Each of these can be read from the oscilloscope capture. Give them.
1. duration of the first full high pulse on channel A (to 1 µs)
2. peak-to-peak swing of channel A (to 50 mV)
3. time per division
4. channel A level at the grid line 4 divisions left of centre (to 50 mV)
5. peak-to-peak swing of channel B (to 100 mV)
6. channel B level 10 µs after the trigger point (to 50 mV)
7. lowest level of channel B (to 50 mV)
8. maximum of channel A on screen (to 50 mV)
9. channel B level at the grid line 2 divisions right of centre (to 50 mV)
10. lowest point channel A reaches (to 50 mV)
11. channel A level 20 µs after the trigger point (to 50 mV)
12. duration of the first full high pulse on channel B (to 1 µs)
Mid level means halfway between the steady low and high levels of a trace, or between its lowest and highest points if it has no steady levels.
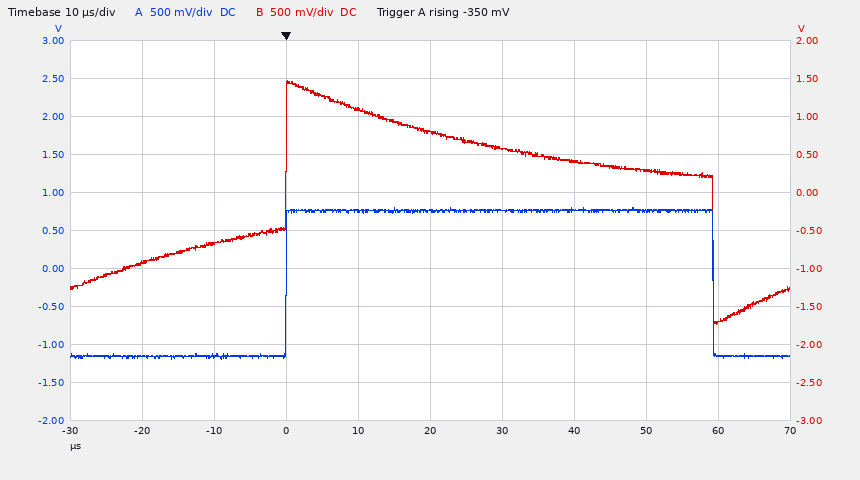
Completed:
59 µs
2.00 V
10 µs
-1.15 V
3.20 V
1.10 V
-1.75 V
800 mV
400 mV
-1.20 V
750 mV
59 µs
